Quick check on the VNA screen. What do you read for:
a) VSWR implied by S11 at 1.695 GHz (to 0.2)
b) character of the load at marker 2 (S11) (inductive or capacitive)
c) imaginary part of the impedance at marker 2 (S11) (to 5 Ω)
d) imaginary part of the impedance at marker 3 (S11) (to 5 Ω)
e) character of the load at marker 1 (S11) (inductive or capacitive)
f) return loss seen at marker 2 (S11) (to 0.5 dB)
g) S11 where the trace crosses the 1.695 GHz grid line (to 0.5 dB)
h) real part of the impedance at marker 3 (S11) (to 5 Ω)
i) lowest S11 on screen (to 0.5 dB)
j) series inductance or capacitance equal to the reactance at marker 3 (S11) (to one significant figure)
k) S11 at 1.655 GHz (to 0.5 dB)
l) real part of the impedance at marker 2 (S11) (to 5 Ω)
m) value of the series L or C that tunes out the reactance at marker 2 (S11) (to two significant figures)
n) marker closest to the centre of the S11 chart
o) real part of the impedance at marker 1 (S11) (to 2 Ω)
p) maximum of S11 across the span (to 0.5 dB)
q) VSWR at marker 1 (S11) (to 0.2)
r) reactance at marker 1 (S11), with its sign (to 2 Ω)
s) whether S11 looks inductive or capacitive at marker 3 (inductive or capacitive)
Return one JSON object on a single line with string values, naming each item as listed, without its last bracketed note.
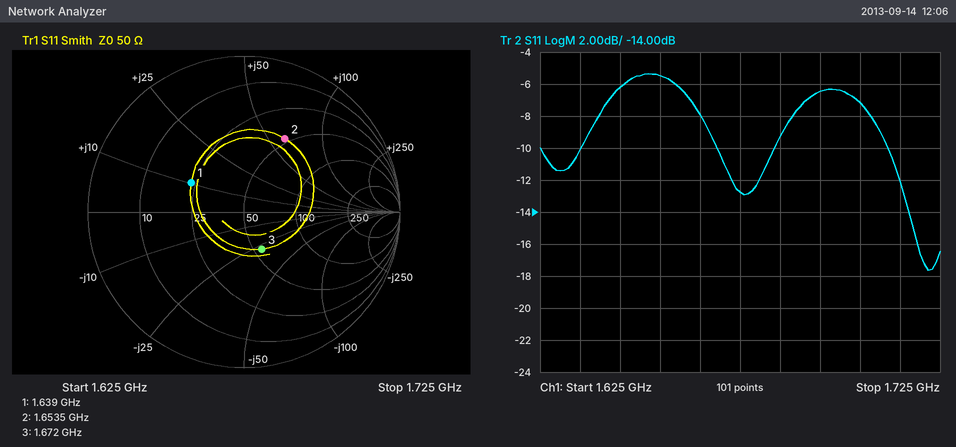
{"VSWR implied by S11 at 1.695 GHz": "2.8", "character of the load at marker 2 (S11)": "inductive", "imaginary part of the impedance at marker 2 (S11)": "+60 Ω", "imaginary part of the impedance at marker 3 (S11)": "-30 Ω", "character of the load at marker 1 (S11)": "inductive", "return loss seen at marker 2 (S11)": "5.5 dB", "S11 where the trace crosses the 1.695 GHz grid line": "-6.5 dB", "real part of the impedance at marker 3 (S11)": "55 Ω", "lowest S11 on screen": "-17.5 dB", "series inductance or capacitance equal to the reactance at marker 3 (S11)": "3 pF", "S11 at 1.655 GHz": "-5.5 dB", "real part of the impedance at marker 2 (S11)": "45 Ω", "value of the series L or C that tunes out the reactance at marker 2 (S11)": "1.6 pF", "marker closest to the centre of the S11 chart": "marker 3", "real part of the impedance at marker 1 (S11)": "24 Ω", "maximum of S11 across the span": "-5.5 dB", "VSWR at marker 1 (S11)": "2.2", "reactance at marker 1 (S11), with its sign": "+10 Ω", "whether S11 looks inductive or capacitive at marker 3": "capacitive"}
